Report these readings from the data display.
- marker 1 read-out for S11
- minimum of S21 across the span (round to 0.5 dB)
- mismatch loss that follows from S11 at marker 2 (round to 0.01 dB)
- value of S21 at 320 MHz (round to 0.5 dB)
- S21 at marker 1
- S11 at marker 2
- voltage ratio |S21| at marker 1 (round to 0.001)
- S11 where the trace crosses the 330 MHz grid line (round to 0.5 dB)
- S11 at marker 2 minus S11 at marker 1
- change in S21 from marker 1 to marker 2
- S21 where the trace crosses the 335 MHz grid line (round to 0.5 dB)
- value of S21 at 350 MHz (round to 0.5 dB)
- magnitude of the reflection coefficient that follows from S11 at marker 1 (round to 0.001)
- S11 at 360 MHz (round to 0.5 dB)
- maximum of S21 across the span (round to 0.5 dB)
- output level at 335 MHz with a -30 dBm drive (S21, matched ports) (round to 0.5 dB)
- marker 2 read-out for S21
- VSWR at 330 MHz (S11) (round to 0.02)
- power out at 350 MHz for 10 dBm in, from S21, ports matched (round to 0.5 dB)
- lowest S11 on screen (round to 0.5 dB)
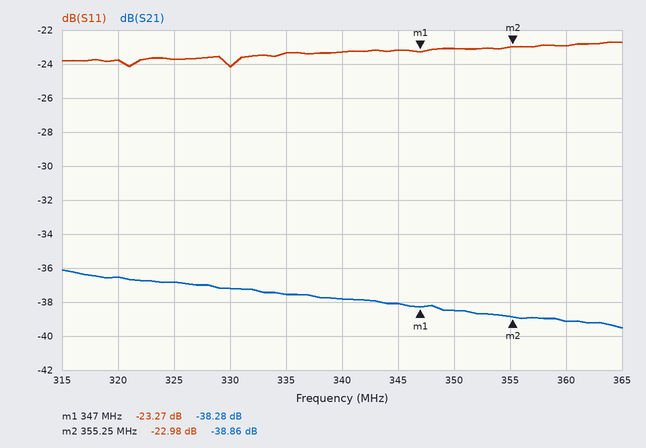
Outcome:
-23.27 dB
-39.5 dB
0.02 dB
-36.5 dB
-38.28 dB
-22.98 dB
0.012
-24.0 dB
0.29 dB
-0.58 dB
-37.5 dB
-38.5 dB
0.069
-23.0 dB
-36.0 dB
-67.5 dBm
-38.86 dB
1.14
-28.5 dBm
-24.0 dB
